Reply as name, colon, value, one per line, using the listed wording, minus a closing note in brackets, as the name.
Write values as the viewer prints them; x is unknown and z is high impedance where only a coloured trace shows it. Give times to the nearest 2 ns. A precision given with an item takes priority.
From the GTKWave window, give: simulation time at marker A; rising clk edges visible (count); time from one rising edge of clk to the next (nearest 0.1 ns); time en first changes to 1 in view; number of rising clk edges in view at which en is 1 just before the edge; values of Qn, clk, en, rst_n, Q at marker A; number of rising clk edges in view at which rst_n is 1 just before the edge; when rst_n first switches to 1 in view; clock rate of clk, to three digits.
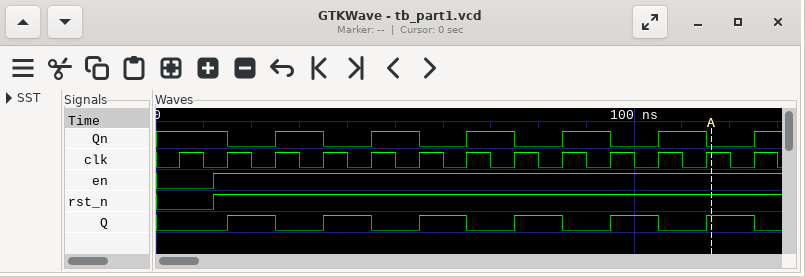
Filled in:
simulation time at marker A: 116 ns
rising clk edges visible: 13
time from one rising edge of clk to the next: 10 ns
time en first changes to 1 in view: 12 ns
number of rising clk edges in view at which en is 1 just before the edge: 12
values of Qn, clk, en, rst_n, Q at marker A: Qn=0, clk=1, en=1, rst_n=1, Q=1
number of rising clk edges in view at which rst_n is 1 just before the edge: 12
when rst_n first switches to 1 in view: 12 ns
clock rate of clk, to three digits: 100 MHz
